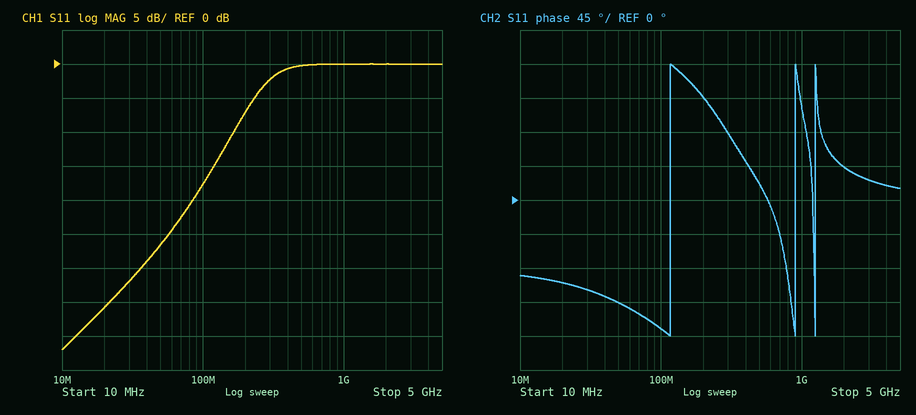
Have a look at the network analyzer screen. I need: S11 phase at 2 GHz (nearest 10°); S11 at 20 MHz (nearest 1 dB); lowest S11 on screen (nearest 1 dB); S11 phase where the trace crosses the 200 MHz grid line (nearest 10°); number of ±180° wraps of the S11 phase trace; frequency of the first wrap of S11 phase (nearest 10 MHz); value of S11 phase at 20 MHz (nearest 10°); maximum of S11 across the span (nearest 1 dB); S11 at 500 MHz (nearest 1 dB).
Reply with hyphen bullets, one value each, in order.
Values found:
- 40°
- -36 dB
- -42 dB
- 140°
- 3
- 120 MHz
- -110°
- 0 dB
- 0 dB
